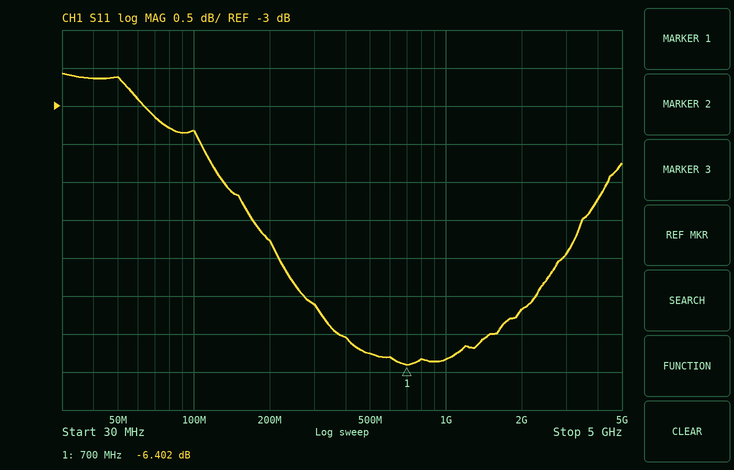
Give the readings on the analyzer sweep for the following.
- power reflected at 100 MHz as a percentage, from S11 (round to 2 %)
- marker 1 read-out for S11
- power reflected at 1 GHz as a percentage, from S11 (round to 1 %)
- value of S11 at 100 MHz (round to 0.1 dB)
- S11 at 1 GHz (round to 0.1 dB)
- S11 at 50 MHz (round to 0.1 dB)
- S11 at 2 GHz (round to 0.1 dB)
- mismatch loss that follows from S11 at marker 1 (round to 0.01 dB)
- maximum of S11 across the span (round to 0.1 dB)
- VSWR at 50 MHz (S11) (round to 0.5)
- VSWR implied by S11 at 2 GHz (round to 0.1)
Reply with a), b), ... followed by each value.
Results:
a) 46 %
b) -6.402 dB
c) 23 %
d) -3.3 dB
e) -6.3 dB
f) -2.6 dB
g) -5.7 dB
h) 1.13 dB
i) -2.6 dB
j) 6.5
k) 3.2
